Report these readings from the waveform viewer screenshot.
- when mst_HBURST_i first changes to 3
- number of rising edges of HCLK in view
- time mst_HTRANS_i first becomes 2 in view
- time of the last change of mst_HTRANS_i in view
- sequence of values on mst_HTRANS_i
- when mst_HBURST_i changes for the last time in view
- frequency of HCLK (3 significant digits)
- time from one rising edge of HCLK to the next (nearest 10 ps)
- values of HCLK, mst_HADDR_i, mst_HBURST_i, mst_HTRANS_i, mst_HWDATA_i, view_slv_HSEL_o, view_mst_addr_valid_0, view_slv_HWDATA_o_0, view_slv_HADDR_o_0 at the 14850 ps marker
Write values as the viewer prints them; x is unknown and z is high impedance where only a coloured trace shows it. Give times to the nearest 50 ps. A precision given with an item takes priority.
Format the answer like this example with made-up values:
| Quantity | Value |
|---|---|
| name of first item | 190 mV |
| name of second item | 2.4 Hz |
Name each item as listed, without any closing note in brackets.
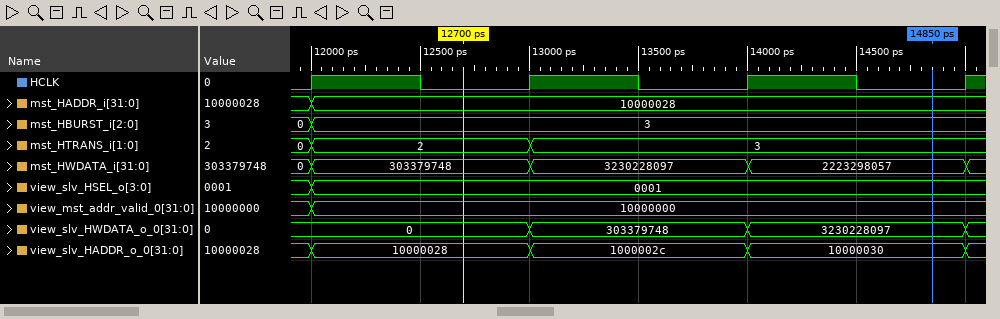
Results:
| Quantity | Value |
|---|---|
| when mst_HBURST_i first changes to 3 | 12000 ps |
| number of rising edges of HCLK in view | 4 |
| time mst_HTRANS_i first becomes 2 in view | 12000 ps |
| time of the last change of mst_HTRANS_i in view | 13000 ps |
| sequence of values on mst_HTRANS_i | 0, 2, 3 |
| when mst_HBURST_i changes for the last time in view | 12000 ps |
| frequency of HCLK | 1.00 GHz |
| time from one rising edge of HCLK to the next | 1000 ps |
| values of HCLK, mst_HADDR_i, mst_HBURST_i, mst_HTRANS_i, mst_HWDATA_i, view_slv_HSEL_o, view_mst_addr_valid_0, view_slv_HWDATA_o_0, view_slv_HADDR_o_0 at the 14850 ps marker | HCLK=0, mst_HADDR_i=10000028, mst_HBURST_i=3, mst_HTRANS_i=3, mst_HWDATA_i=2223298057, view_slv_HSEL_o=0001, view_mst_addr_valid_0=10000000, view_slv_HWDATA_o_0=3230228097, view_slv_HADDR_o_0=10000030 |
